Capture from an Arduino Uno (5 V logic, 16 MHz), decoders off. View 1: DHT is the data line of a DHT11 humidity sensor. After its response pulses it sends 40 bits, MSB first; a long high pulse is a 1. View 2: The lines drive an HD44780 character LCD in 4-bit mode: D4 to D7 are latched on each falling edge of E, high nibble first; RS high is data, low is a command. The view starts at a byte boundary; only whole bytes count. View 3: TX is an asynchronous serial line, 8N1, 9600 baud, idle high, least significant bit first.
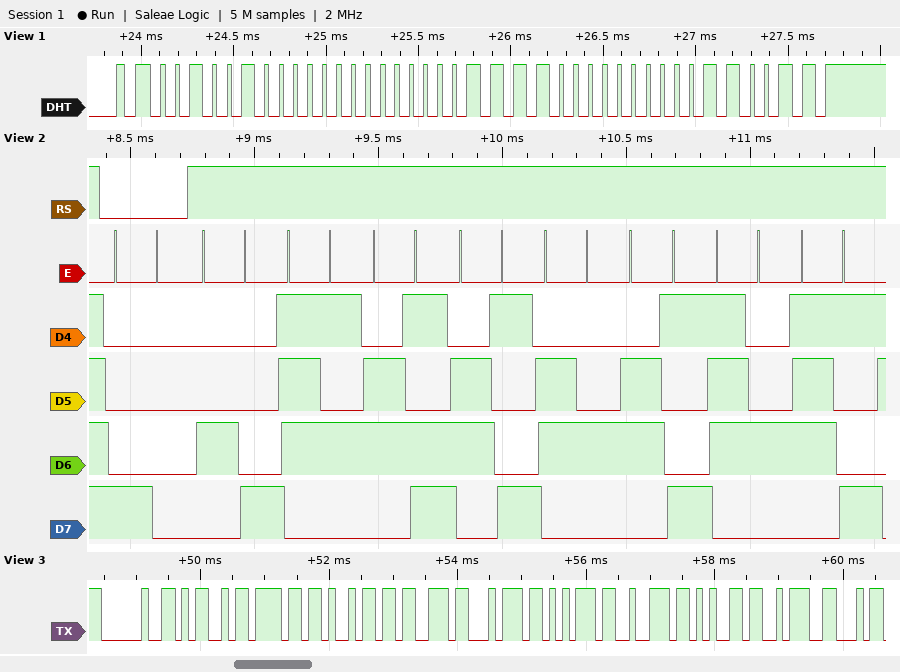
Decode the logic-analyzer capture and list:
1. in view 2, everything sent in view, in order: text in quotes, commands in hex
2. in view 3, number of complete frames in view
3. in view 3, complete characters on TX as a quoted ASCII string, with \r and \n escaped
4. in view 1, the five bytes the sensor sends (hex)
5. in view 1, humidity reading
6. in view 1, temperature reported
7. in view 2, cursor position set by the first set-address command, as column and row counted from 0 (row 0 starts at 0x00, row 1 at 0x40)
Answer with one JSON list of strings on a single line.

["0x80 \"Humidity\"", "10", "\" Moisture:\"", "24 00 0F 00 33", "36 %", "15.0 °C", "column 0, row 0"]
